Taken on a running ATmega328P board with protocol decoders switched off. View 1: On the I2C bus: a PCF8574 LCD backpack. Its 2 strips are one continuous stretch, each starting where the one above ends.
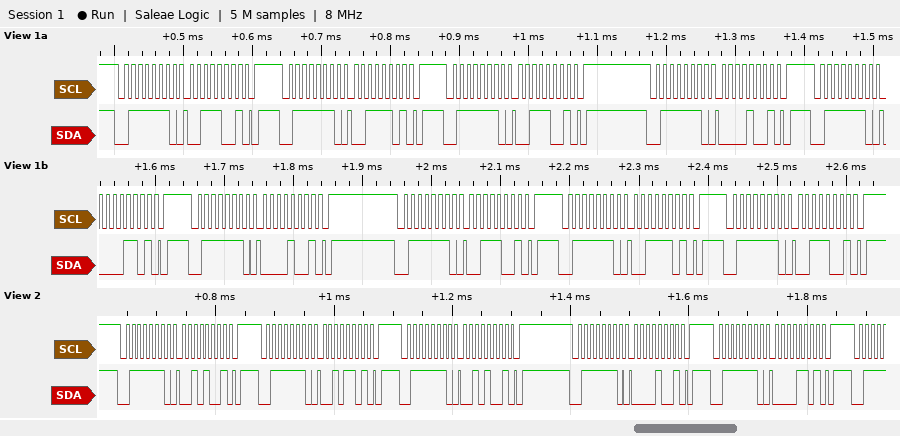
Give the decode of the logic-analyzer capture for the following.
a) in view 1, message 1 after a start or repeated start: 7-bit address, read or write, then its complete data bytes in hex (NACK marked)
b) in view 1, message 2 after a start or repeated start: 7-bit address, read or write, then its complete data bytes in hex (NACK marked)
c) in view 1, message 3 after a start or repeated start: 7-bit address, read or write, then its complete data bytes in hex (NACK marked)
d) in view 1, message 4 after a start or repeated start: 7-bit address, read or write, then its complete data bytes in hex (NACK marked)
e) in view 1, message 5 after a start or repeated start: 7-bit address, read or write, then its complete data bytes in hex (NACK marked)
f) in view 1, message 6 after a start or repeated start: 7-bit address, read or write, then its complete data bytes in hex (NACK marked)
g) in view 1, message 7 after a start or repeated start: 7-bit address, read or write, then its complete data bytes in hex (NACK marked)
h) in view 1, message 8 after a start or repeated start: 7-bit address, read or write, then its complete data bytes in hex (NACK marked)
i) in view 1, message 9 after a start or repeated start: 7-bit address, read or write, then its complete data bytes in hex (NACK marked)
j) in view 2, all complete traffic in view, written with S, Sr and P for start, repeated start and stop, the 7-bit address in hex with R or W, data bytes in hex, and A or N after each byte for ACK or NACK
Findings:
0x3F write: 39
0x3F write: 3D
0x3F write: 39
0x3F write: 09
0x3F write: 0D
0x3F write: 09
0x3F write: 39
0x3F write: 3D
0x3F write: 39
S 3FW A 29 A P S 3FW A 2D A P S 3FW A 29 A P S 3FW A 09 A P S 3FW A 0D A P
